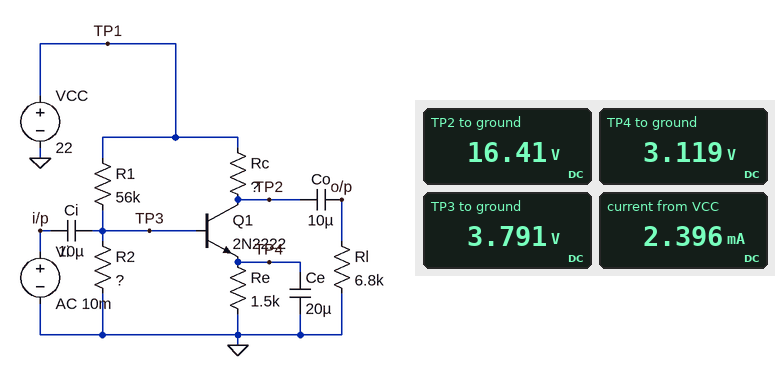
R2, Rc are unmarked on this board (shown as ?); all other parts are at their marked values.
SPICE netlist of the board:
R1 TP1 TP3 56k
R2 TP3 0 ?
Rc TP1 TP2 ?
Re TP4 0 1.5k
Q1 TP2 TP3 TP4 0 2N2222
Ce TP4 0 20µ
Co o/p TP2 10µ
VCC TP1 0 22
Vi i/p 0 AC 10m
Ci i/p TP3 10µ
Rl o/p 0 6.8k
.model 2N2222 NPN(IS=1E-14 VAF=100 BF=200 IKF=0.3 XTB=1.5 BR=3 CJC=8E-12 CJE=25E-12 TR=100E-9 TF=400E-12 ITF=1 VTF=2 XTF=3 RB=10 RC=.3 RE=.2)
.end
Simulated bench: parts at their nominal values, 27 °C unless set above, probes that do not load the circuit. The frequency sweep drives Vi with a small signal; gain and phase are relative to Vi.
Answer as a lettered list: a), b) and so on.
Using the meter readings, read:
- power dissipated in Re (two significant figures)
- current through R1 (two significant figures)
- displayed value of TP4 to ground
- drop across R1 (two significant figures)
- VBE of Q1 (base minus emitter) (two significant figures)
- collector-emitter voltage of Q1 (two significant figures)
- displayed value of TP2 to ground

a) 6.5 mW
b) 330 µA
c) 3.119 V
d) 18 V
e) 670 mV
f) 13 V
g) 16.41 V
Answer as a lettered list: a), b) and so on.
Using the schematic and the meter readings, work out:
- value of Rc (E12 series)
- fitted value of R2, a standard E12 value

a) 2.7 kΩ
b) 12 kΩ
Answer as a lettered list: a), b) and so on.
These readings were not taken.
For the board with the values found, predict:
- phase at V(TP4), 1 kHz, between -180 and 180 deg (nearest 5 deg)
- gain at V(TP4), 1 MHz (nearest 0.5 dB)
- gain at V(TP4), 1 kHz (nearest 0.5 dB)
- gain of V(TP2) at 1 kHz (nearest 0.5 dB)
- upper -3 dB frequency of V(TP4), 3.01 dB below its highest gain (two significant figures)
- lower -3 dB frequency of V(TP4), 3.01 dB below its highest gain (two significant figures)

a) -60 deg
b) -64.5 dB
c) -6.0 dB
d) 42.0 dB
e) 620 Hz
f) 1.6 Hz
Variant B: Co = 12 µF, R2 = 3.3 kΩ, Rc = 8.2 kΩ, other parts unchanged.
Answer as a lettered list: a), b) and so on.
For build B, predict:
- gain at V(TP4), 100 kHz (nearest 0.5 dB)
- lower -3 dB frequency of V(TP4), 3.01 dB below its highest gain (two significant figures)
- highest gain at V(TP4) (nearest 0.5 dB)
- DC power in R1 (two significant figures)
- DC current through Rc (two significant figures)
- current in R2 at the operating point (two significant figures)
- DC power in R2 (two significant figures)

a) -58.5 dB
b) 4.7 Hz
c) -1.0 dB
d) 7.7 mW
e) 390 µA
f) 370 µA
g) 450 µW
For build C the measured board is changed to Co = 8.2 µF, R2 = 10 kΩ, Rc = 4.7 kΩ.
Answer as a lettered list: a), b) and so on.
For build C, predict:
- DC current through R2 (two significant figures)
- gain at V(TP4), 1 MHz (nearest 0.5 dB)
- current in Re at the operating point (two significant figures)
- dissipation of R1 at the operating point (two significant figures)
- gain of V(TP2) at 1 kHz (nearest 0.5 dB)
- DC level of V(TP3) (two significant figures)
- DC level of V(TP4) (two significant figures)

a) 330 µA
b) -66.0 dB
c) 1.7 mA
d) 6.3 mW
e) 44.0 dB
f) 3.3 V
g) 2.6 V
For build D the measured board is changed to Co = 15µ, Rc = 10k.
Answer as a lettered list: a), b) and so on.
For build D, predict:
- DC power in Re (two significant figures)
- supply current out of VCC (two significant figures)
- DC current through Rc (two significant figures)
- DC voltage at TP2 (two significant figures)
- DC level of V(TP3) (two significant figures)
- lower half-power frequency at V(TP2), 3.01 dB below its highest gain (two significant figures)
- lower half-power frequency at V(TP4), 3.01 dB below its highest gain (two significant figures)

a) 5.6 mW
b) 2.2 mA
c) 1.9 mA
d) 3.0 V
e) 3.6 V
f) 400 Hz
g) 5.1 Hz
